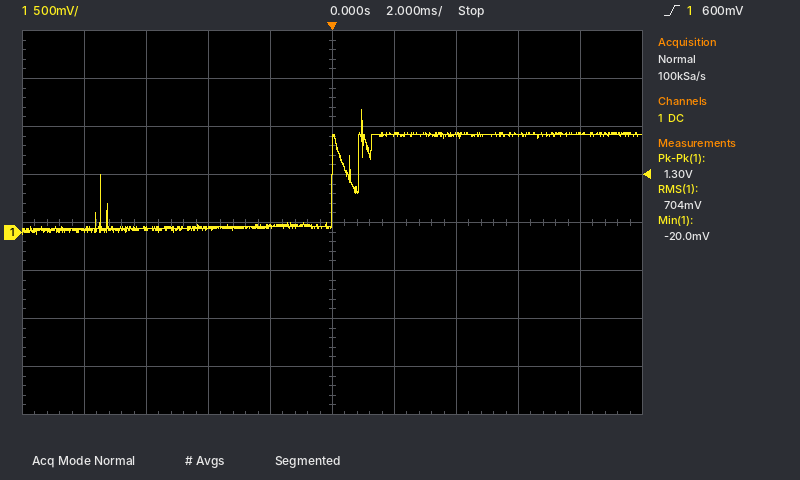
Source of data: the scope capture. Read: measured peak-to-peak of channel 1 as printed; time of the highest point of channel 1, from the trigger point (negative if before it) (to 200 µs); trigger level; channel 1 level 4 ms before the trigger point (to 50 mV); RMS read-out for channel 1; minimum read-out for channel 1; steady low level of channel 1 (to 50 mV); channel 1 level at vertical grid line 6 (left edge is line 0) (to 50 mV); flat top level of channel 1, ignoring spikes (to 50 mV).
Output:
1.30 V
+1.0 ms
600 mV
50 mV
704 mV
-20.0 mV
50 mV
1.00 V
1.00 V
